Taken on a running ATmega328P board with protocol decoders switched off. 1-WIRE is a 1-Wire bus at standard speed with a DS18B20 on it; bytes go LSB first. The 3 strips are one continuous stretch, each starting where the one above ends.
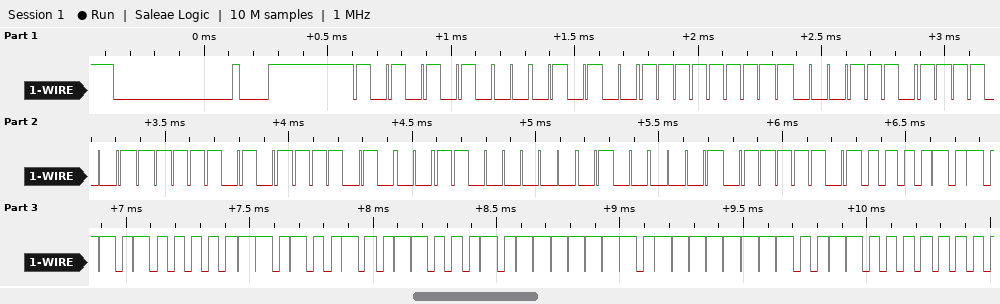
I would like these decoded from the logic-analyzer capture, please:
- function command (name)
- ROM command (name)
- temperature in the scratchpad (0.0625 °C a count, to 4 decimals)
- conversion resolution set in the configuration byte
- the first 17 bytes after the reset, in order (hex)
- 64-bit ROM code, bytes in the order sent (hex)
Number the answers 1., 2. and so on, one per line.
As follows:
1. Read Scratchpad
2. Match ROM
3. 85.0000 °C
4. 12 bits
5. 55 28 FF 71 CF AF 17 03 82 BE 50 05 4B 46 7F FF 0C
6. 28 FF 71 CF AF 17 03 82
